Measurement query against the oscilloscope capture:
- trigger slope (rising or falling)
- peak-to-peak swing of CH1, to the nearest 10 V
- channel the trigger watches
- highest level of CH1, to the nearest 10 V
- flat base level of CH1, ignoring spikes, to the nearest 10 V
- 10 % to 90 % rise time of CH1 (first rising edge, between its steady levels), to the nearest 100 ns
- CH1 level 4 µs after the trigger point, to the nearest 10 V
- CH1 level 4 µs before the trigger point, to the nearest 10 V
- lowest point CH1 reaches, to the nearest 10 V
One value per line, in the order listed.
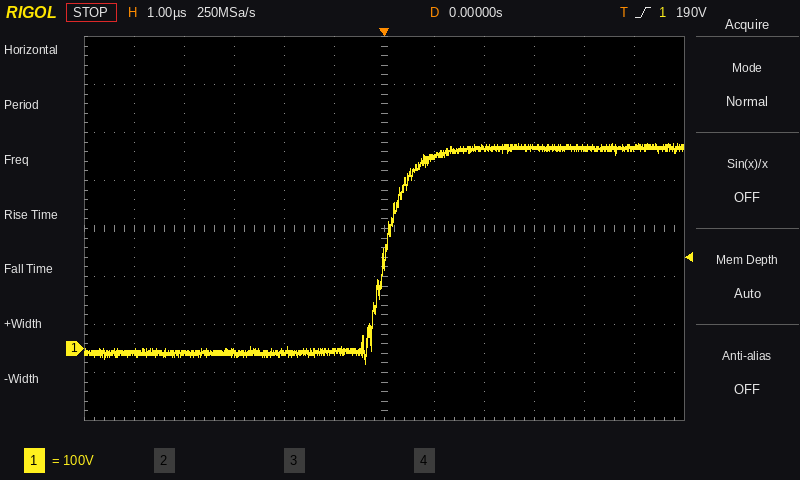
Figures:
rising
460 V
CH1
430 V
-10 V
900 ns
420 V
-10 V
-30 V
